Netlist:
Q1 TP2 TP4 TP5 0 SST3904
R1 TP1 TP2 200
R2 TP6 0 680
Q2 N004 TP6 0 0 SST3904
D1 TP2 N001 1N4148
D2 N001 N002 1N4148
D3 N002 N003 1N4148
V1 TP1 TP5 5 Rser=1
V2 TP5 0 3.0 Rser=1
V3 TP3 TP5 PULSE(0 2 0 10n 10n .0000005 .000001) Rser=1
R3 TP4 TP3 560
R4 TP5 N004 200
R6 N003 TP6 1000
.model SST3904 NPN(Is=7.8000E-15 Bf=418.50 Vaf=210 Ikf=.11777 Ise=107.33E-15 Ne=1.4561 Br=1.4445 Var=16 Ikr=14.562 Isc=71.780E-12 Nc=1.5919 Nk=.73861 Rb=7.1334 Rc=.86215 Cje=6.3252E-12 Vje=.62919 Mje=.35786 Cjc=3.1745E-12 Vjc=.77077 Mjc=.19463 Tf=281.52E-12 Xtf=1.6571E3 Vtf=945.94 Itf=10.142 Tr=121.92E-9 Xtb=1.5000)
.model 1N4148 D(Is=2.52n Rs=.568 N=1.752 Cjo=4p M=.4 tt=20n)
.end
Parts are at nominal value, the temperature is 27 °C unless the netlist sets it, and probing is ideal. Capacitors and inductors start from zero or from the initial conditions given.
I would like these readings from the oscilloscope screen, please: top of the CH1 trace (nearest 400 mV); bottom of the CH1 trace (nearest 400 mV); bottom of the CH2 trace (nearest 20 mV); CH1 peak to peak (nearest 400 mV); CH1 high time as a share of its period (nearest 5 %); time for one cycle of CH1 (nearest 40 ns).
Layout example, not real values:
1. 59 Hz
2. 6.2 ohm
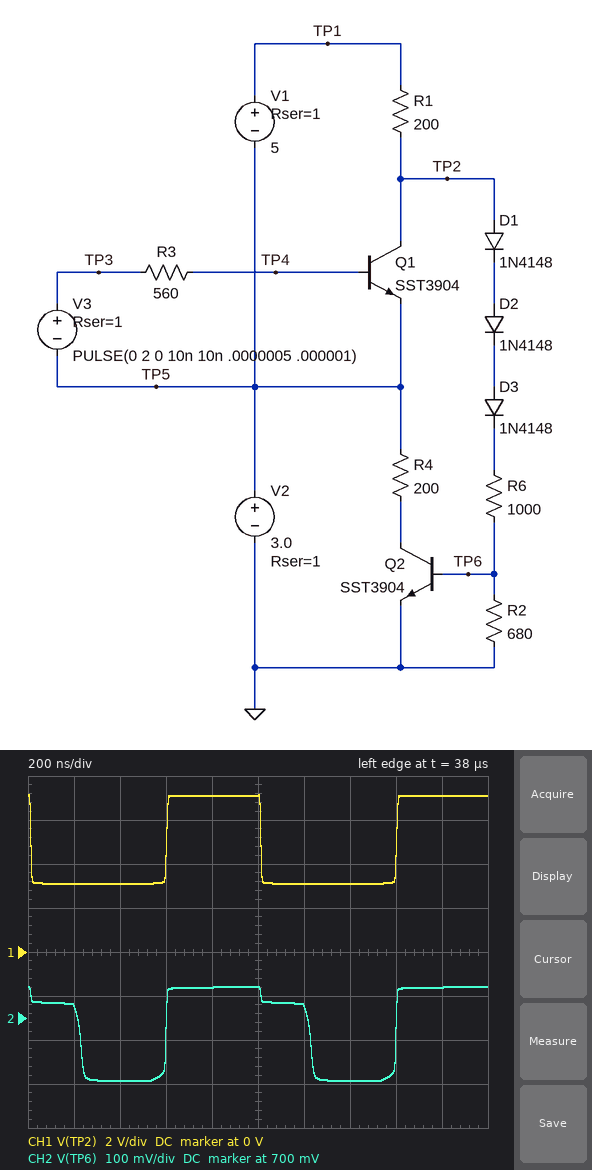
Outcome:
1. 7.2 V
2. 3.2 V
3. 560 mV
4. 4.0 V
5. 40 %
6. 1.00 µs
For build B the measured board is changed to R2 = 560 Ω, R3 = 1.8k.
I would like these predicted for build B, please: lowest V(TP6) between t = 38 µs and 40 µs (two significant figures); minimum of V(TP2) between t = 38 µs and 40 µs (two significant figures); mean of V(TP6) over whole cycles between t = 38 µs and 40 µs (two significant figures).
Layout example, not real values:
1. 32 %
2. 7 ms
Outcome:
1. 500 mV
2. 3.1 V
3. 660 mV
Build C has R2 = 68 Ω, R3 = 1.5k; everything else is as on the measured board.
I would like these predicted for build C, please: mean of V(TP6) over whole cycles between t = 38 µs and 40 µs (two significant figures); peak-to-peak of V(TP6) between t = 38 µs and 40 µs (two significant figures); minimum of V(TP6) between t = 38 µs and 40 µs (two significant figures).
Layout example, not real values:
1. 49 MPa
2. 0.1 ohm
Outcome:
1. 190 mV
2. 240 mV
3. 83 mV
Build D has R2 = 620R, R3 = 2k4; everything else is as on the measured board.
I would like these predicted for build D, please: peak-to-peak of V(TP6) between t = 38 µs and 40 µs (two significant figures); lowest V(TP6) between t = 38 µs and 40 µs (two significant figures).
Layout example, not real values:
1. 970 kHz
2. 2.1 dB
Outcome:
1. 230 mV
2. 540 mV
